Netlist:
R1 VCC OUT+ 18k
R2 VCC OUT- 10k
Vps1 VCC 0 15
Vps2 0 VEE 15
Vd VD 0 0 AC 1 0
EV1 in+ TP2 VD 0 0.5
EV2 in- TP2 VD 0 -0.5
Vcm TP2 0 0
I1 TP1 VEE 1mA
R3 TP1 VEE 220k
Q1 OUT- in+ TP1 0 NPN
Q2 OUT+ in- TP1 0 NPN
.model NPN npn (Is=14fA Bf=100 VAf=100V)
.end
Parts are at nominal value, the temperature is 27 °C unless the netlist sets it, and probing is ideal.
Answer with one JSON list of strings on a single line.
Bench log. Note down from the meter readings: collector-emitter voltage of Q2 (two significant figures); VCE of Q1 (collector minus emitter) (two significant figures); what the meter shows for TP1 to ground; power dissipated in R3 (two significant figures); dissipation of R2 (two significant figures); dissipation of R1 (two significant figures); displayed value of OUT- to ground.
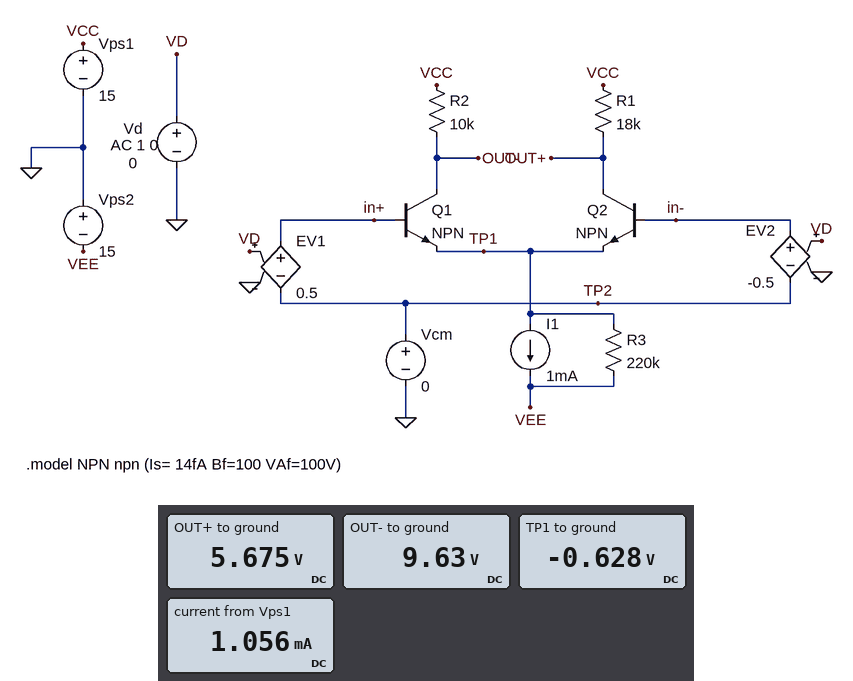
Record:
["6.3 V", "10 V", "-0.628 V", "940 µW", "2.9 mW", "4.8 mW", "9.63 V"]
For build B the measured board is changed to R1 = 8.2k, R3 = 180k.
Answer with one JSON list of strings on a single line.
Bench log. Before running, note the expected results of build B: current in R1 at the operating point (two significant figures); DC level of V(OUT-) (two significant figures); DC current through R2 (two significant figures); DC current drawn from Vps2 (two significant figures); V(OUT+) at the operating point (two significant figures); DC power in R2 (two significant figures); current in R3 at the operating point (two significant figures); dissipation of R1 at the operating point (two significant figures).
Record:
["540 µA", "9.7 V", "530 µA", "1.1 mA", "11 V", "2.8 mW", "80 µA", "2.4 mW"]
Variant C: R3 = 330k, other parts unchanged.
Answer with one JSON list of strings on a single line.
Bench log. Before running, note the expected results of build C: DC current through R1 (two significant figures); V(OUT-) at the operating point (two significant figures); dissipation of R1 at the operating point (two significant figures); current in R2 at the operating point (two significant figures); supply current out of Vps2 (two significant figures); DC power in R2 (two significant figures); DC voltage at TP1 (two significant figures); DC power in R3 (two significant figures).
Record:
["510 µA", "9.7 V", "4.6 mW", "530 µA", "1.0 mA", "2.8 mW", "-630 mV", "630 µW"]
